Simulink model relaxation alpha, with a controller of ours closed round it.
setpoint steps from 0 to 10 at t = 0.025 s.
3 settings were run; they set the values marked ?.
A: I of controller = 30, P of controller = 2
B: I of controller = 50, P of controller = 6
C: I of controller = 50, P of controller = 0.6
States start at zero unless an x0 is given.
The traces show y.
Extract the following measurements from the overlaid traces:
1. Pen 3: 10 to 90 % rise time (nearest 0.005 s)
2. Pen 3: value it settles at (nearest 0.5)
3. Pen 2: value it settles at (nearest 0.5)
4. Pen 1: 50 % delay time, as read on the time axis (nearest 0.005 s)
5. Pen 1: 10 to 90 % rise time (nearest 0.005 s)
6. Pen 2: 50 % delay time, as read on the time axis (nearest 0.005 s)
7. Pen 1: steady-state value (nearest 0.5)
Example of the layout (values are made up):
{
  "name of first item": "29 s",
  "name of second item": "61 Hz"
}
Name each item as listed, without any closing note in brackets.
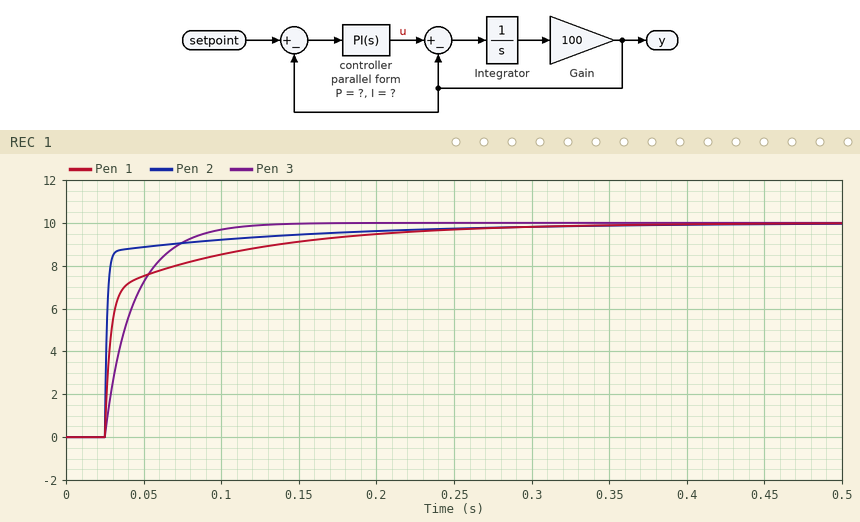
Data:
{
  "Pen 3: 10 to 90 % rise time": "0.045 s",
  "Pen 3: value it settles at": "10.0",
  "Pen 2: value it settles at": "10.0",
  "Pen 1: 50 % delay time, as read on the time axis": "0.030 s",
  "Pen 1: 10 to 90 % rise time": "0.110 s",
  "Pen 2: 50 % delay time, as read on the time axis": "0.025 s",
  "Pen 1: steady-state value": "10.0"
}
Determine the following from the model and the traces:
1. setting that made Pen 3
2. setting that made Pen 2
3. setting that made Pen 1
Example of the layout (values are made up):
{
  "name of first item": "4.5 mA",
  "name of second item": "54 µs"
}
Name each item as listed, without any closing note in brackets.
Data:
{
  "setting that made Pen 3": "C",
  "setting that made Pen 2": "B",
  "setting that made Pen 1": "A"
}
